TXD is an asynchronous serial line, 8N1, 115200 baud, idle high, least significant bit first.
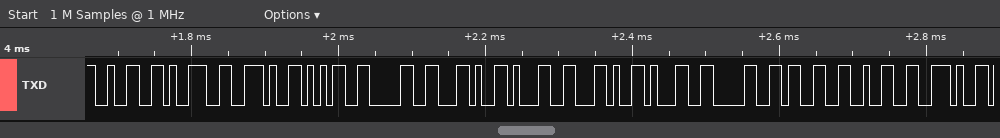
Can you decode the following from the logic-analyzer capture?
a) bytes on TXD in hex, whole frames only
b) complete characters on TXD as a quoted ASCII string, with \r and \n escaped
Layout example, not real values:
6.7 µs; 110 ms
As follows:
32 39 2E 35 30 2C 31 2C 31 30 33 32 2E; "29.50,1,1032."
